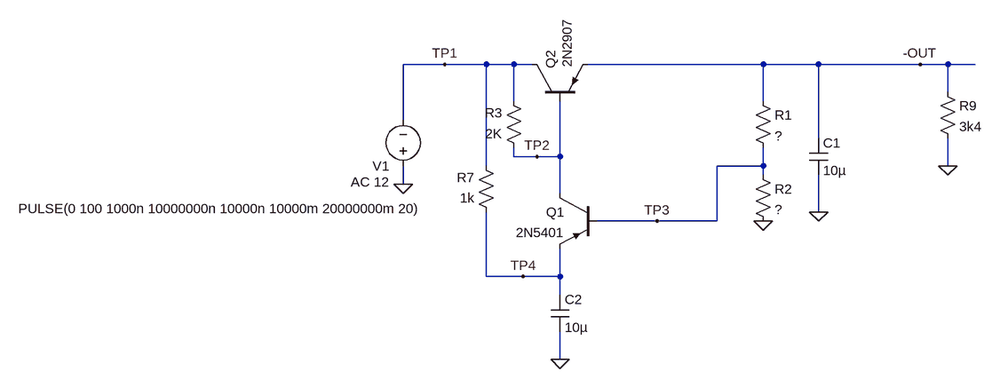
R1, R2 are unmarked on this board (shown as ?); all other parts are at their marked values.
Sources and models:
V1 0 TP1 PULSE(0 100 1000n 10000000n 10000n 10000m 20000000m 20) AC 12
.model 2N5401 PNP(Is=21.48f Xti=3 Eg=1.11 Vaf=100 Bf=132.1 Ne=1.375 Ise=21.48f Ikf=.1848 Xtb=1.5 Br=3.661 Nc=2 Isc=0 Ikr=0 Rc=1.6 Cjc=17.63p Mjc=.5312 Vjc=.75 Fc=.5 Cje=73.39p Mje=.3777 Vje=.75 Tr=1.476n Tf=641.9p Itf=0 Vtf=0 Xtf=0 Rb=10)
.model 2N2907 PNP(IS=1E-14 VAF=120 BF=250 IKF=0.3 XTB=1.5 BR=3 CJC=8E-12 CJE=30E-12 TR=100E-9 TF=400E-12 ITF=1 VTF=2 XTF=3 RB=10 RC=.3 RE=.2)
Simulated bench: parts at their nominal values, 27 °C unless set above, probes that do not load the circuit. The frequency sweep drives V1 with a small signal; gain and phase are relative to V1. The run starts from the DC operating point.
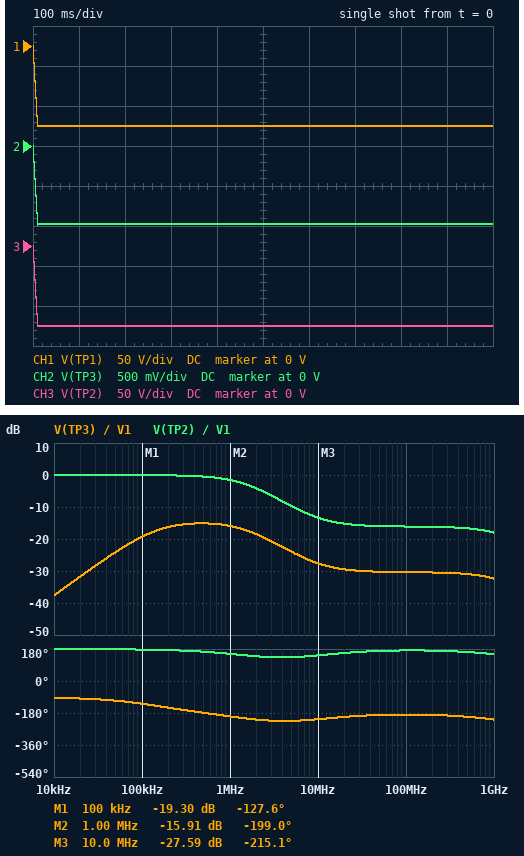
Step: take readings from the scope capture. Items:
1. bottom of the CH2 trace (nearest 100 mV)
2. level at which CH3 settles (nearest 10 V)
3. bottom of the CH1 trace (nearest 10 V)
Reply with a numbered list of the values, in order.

1. -1.0 V
2. -100 V
3. -100 V
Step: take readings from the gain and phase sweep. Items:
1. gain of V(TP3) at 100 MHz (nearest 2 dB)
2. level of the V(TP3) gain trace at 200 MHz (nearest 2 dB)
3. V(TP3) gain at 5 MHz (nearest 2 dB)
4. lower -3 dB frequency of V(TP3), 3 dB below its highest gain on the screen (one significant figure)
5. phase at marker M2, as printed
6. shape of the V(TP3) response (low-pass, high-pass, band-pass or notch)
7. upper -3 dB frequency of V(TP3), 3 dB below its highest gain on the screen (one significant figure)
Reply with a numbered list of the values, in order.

1. -30 dB
2. -30 dB
3. -24 dB
4. 100 kHz
5. -199.0 deg
6. band-pass
7. 2 MHz
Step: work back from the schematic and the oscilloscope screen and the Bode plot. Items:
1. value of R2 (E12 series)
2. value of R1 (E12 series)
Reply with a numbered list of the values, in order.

1. 12 kΩ
2. 1.2 MΩ
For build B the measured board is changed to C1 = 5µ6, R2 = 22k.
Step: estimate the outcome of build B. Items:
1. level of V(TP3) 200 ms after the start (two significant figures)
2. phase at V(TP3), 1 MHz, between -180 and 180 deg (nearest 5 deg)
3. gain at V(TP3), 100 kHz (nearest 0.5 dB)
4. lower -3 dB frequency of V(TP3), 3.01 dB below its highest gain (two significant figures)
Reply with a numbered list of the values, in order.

1. -1.8 V
2. 155 deg
3. -16.5 dB
4. 73 kHz
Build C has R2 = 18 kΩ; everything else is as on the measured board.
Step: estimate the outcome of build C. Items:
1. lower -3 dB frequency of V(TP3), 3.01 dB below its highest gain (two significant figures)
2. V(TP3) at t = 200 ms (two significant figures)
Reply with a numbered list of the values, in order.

1. 88 kHz
2. -1.5 V
